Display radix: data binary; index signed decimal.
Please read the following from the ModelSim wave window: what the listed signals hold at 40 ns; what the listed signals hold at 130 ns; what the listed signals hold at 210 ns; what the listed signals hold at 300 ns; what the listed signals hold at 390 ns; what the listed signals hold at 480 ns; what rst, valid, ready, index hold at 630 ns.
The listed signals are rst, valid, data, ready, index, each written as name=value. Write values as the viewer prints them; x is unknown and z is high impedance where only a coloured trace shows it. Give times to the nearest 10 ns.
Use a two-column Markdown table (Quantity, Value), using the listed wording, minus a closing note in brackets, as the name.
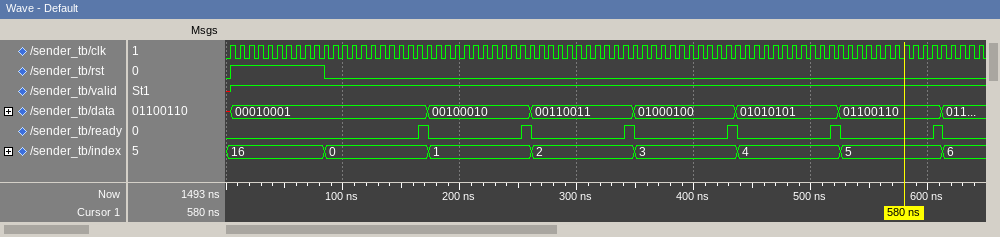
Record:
| Quantity | Value |
|---|---|
| what the listed signals hold at 40 ns | rst=1, valid=1, data=00010001, ready=0, index=16 |
| what the listed signals hold at 130 ns | rst=0, valid=1, data=00010001, ready=0, index=0 |
| what the listed signals hold at 210 ns | rst=0, valid=1, data=00100010, ready=0, index=1 |
| what the listed signals hold at 300 ns | rst=0, valid=1, data=00110011, ready=0, index=2 |
| what the listed signals hold at 390 ns | rst=0, valid=1, data=01000100, ready=0, index=3 |
| what the listed signals hold at 480 ns | rst=0, valid=1, data=01010101, ready=0, index=4 |
| what rst, valid, ready, index hold at 630 ns | rst=0, valid=1, ready=0, index=6 |
